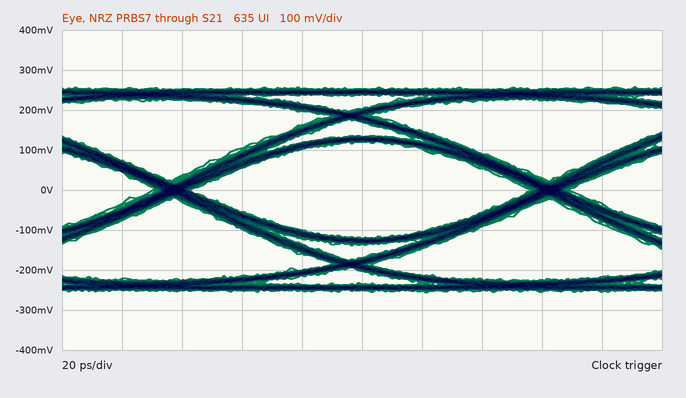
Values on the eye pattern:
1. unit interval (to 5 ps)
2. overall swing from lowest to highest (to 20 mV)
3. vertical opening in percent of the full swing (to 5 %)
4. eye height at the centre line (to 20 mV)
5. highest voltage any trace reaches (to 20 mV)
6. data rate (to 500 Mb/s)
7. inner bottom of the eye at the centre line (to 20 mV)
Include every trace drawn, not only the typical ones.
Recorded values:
125 ps
520 mV
45 %
240 mV
260 mV
8.0 Gb/s
-120 mV
